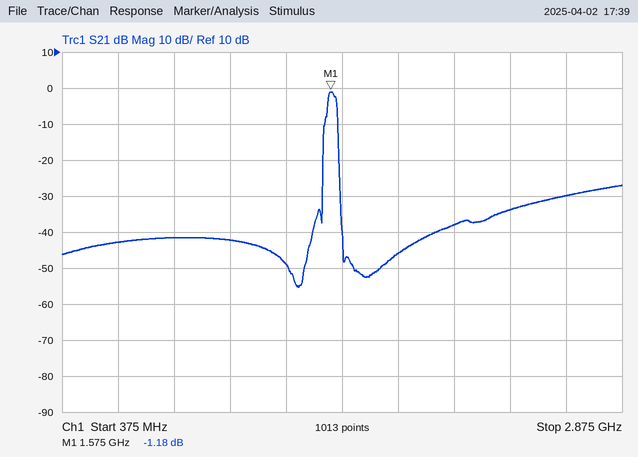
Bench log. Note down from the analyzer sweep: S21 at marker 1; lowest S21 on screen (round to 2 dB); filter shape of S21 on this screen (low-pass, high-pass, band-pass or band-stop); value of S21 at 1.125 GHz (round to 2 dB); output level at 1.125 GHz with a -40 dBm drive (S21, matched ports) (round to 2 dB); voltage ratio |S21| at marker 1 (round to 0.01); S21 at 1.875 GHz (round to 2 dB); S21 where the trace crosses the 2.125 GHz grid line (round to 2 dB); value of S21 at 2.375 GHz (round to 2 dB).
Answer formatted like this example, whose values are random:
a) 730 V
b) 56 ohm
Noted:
a) -1.18 dB
b) -56 dB
c) band-pass
d) -42 dB
e) -82 dBm
f) 0.87
g) -46 dB
h) -38 dB
i) -34 dB
